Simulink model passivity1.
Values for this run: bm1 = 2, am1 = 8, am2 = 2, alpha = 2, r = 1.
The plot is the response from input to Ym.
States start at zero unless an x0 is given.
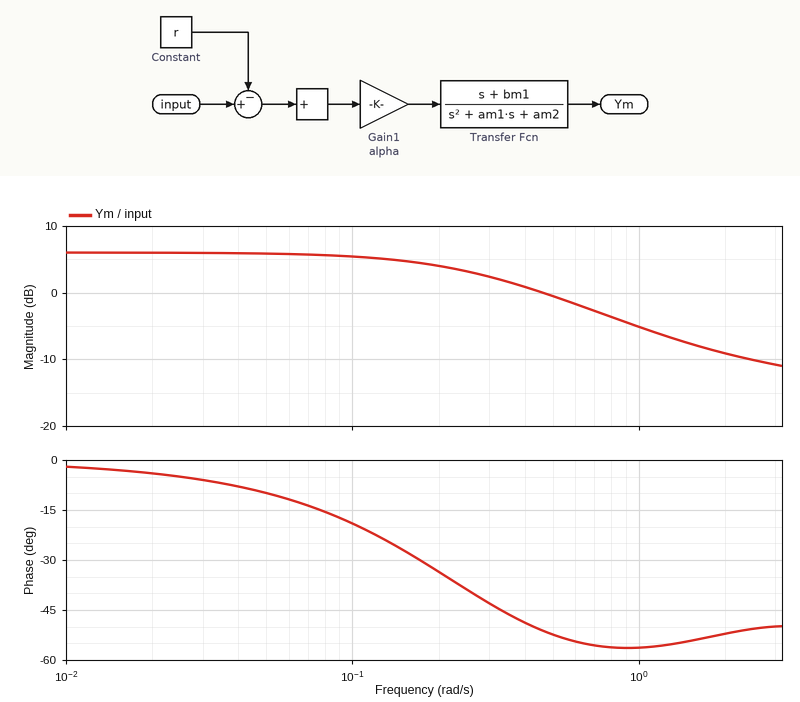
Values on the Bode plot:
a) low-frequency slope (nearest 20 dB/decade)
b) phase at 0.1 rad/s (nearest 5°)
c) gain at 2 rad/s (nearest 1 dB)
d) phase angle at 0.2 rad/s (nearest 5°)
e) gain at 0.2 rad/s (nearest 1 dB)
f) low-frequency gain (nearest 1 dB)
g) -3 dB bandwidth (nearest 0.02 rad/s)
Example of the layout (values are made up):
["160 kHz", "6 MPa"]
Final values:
["0 dB/decade", "-20°", "-9 dB", "-35°", "4 dB", "6 dB", "0.26 rad/s"]
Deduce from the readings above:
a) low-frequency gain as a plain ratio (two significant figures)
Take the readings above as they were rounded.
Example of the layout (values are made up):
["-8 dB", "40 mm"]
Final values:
["2.0"]
